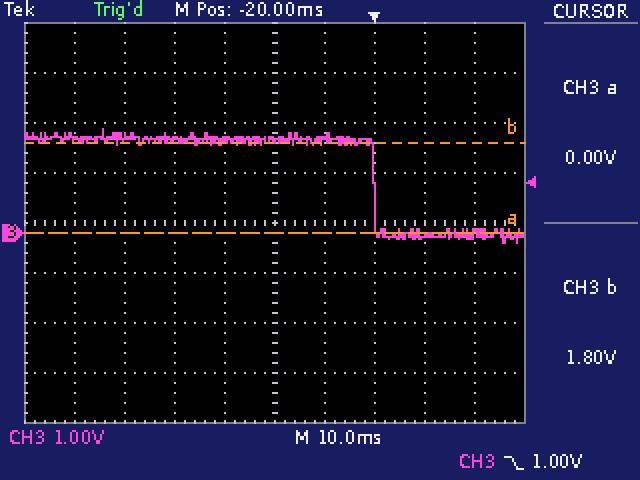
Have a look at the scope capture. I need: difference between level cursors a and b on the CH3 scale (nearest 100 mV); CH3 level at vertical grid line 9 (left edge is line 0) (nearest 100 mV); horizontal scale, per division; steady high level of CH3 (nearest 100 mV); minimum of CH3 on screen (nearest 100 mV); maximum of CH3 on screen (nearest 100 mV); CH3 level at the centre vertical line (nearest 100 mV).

1.8 V
0.0 V
10 ms
1.9 V
-200 mV
2.1 V
1.9 V
